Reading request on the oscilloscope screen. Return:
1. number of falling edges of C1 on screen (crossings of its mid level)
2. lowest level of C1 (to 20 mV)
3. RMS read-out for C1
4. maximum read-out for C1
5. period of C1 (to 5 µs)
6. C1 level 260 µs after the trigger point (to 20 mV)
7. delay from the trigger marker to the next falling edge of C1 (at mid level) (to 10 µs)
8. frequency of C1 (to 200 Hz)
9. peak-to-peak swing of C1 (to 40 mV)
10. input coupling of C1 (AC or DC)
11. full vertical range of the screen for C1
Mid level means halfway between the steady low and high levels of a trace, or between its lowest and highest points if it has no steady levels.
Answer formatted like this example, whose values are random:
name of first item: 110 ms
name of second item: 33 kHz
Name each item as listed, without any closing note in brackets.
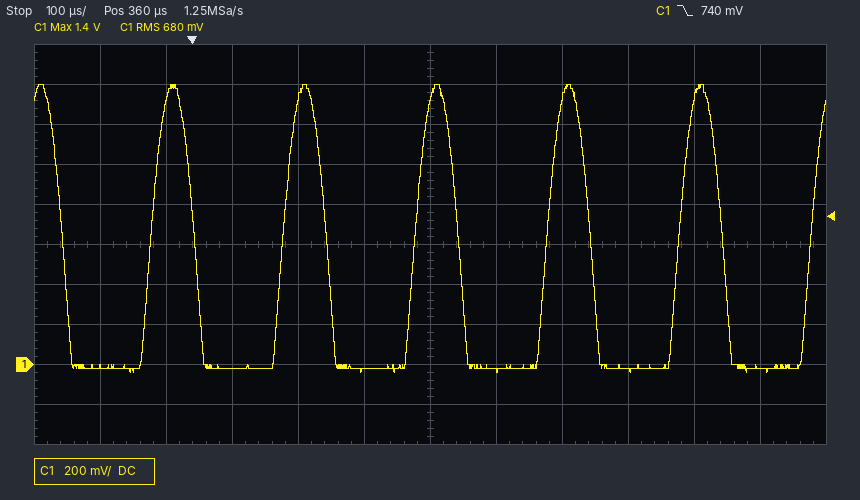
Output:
number of falling edges of C1 on screen: 6
lowest level of C1: -40 mV
RMS read-out for C1: 680 mV
maximum read-out for C1: 1.4 V
period of C1: 200 µs
C1 level 260 µs after the trigger point: -20 mV
delay from the trigger marker to the next falling edge of C1 (at mid level): 200 µs
frequency of C1: 5.0 kHz
peak-to-peak swing of C1: 1.44 V
input coupling of C1: DC
full vertical range of the screen for C1: 2 V
